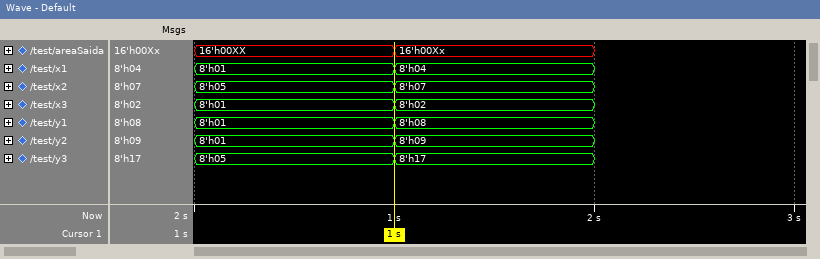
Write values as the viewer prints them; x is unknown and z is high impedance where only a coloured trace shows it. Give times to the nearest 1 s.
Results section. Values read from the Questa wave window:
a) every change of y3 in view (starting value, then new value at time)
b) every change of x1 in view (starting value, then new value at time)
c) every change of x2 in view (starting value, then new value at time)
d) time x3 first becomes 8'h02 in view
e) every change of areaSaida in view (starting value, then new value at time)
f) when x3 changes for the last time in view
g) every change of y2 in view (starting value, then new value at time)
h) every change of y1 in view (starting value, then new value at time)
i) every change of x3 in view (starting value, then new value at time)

8'h05, 8'h17 at 1 s
8'h01, 8'h04 at 1 s
8'h05, 8'h07 at 1 s
1 s
16'h00XX, 16'h00Xx at 1 s
1 s
8'h01, 8'h09 at 1 s
8'h01, 8'h08 at 1 s
8'h01, 8'h02 at 1 s
